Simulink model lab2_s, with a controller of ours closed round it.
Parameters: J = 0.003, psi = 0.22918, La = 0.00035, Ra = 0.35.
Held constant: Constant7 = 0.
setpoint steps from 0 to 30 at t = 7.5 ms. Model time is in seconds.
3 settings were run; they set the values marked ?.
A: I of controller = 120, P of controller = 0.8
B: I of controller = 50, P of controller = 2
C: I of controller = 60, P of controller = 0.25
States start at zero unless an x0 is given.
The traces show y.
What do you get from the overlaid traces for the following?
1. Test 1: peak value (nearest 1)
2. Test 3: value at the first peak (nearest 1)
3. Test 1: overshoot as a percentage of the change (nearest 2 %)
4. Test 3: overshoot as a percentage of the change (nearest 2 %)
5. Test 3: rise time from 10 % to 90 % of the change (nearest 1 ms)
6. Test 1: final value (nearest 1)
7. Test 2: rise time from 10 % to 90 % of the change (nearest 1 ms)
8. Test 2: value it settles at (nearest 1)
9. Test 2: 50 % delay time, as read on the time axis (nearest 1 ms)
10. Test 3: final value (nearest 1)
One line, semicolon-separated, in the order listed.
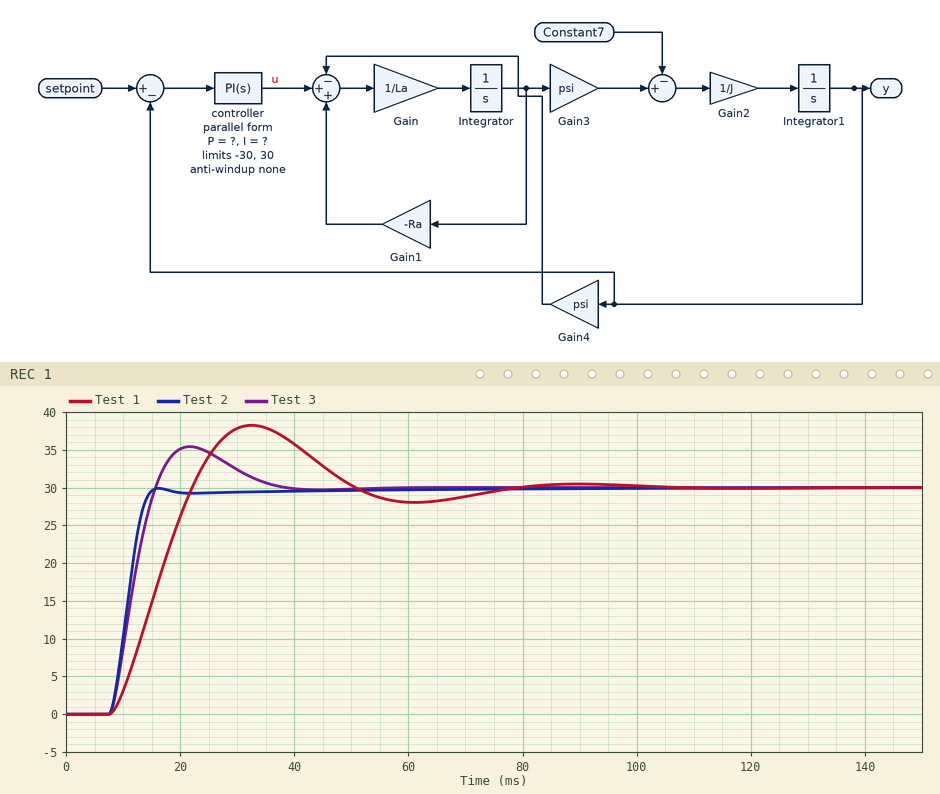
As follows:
38; 35; 28 %; 18 %; 6 ms; 30; 5 ms; 30; 11 ms; 30
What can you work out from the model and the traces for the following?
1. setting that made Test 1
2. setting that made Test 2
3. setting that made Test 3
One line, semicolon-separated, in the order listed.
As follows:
C; B; A
